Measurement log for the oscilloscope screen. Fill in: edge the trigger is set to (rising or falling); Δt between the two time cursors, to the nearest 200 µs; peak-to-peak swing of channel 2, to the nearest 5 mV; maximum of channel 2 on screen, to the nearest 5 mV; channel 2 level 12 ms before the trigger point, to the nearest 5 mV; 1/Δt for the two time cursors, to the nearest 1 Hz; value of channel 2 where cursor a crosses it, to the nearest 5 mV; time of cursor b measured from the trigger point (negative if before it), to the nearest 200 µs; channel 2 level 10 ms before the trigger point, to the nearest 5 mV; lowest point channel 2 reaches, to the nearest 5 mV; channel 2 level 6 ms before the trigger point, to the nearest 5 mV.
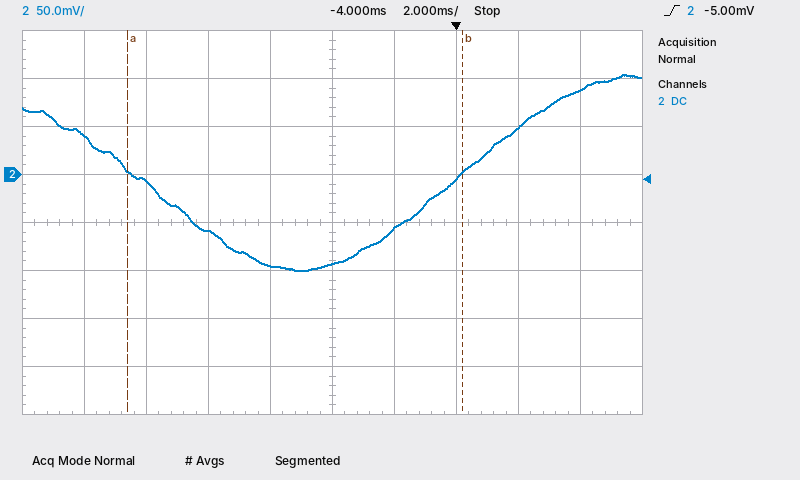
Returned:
rising
10.8 ms
205 mV
105 mV
40 mV
93 Hz
5 mV
+200 µs
-5 mV
-100 mV
-95 mV
